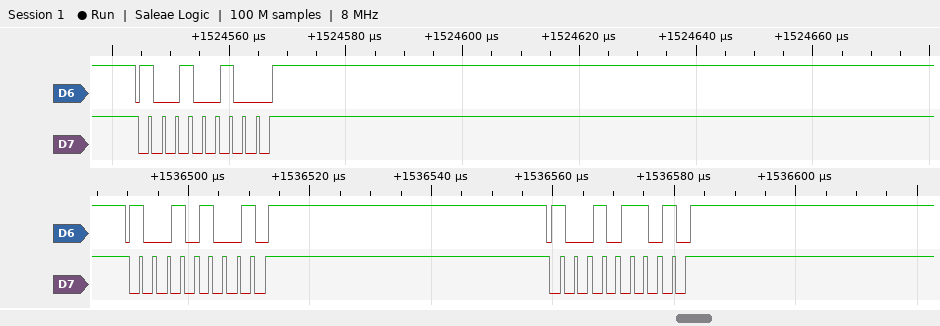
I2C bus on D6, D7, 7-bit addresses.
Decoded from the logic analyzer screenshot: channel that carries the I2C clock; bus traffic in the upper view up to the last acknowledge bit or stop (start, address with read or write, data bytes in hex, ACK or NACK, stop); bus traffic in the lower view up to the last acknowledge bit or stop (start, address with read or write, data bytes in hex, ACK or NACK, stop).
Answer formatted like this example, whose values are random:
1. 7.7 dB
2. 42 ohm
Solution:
1. D7
2. start, address 49 write ACK, stop
3. start, address 4A write NACK, stop, start, address 4B write NACK, stop
